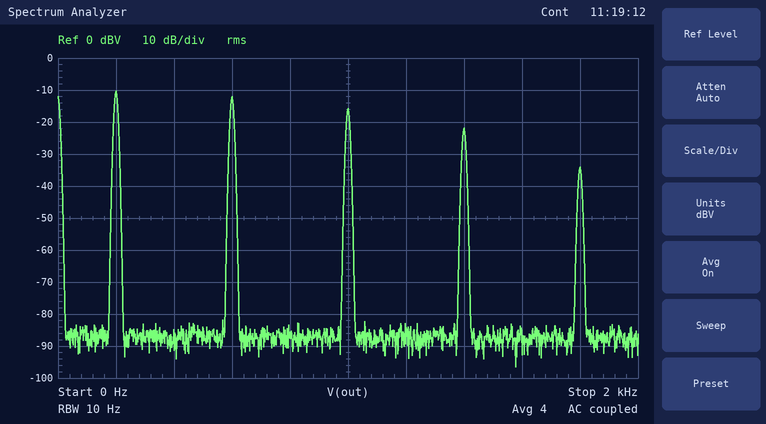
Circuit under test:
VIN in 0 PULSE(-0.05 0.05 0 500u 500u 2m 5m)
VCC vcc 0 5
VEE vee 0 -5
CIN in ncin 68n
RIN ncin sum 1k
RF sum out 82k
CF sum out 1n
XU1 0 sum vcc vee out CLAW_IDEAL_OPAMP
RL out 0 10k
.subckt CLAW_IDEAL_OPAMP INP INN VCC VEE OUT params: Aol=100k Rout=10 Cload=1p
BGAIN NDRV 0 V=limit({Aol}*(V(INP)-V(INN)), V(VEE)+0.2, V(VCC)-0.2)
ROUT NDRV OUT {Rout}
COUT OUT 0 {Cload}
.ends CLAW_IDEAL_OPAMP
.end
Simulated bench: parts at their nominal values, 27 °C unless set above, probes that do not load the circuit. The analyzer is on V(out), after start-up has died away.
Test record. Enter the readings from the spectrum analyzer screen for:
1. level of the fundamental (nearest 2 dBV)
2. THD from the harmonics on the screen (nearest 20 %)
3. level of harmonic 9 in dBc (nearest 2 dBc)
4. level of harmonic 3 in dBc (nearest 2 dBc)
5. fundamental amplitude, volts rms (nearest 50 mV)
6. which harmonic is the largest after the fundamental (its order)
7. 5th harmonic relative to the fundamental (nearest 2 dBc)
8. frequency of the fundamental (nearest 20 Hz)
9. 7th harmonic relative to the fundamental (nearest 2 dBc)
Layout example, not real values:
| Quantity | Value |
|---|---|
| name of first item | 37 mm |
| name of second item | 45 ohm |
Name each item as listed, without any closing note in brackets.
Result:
| Quantity | Value |
|---|---|
| level of the fundamental | -10 dBV |
| THD from the harmonics on the screen | 100 % |
| level of harmonic 9 in dBc | -24 dBc |
| level of harmonic 3 in dBc | -2 dBc |
| fundamental amplitude, volts rms | 300 mV |
| which harmonic is the largest after the fundamental | 3 |
| 5th harmonic relative to the fundamental | -6 dBc |
| frequency of the fundamental | 200 Hz |
| 7th harmonic relative to the fundamental | -12 dBc |
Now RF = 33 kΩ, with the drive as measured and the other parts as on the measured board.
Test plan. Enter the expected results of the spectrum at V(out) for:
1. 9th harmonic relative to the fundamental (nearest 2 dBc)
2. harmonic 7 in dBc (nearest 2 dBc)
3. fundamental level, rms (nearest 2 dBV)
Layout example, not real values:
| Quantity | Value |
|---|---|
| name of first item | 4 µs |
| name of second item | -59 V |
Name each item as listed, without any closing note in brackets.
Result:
| Quantity | Value |
|---|---|
| 9th harmonic relative to the fundamental | -22 dBc |
| harmonic 7 in dBc | -10 dBc |
| fundamental level, rms | -18 dBV |
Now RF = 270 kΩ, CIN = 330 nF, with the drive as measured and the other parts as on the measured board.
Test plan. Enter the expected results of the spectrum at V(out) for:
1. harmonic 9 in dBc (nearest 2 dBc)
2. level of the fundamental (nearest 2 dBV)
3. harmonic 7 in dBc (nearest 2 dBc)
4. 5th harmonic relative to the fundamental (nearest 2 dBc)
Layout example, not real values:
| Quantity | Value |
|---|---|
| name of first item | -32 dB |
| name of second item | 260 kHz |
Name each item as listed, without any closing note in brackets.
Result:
| Quantity | Value |
|---|---|
| harmonic 9 in dBc | -26 dBc |
| level of the fundamental | 12 dBV |
| harmonic 7 in dBc | -24 dBc |
| 5th harmonic relative to the fundamental | -18 dBc |
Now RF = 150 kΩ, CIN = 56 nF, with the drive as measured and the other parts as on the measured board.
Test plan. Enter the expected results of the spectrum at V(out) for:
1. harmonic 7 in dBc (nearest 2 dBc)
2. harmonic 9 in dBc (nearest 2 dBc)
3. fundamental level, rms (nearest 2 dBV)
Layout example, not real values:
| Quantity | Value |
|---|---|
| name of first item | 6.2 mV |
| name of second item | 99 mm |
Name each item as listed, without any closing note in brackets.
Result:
| Quantity | Value |
|---|---|
| harmonic 7 in dBc | -14 dBc |
| harmonic 9 in dBc | -26 dBc |
| fundamental level, rms | -6 dBV |
